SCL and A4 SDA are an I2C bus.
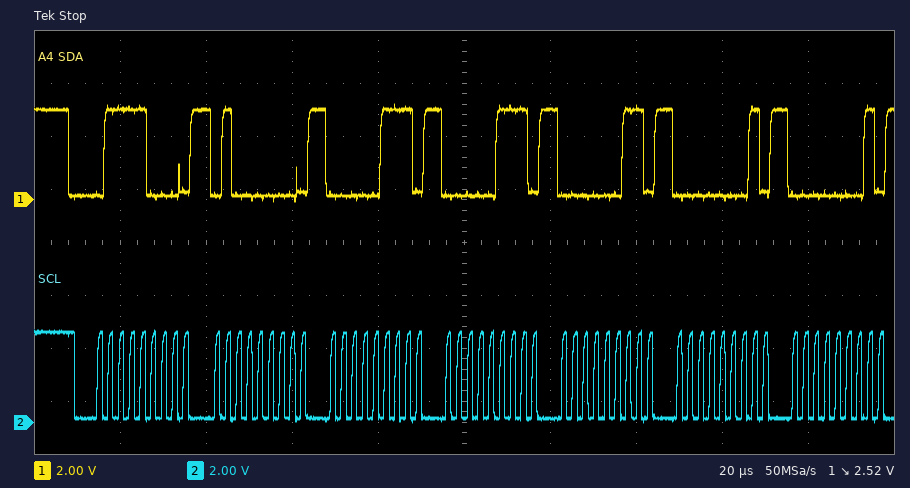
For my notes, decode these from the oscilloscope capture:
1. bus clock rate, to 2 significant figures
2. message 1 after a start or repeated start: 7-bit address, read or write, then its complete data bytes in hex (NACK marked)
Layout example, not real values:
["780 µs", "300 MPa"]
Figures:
["400 kHz", "0x3C write: 40 07 07 03 01 01"]
